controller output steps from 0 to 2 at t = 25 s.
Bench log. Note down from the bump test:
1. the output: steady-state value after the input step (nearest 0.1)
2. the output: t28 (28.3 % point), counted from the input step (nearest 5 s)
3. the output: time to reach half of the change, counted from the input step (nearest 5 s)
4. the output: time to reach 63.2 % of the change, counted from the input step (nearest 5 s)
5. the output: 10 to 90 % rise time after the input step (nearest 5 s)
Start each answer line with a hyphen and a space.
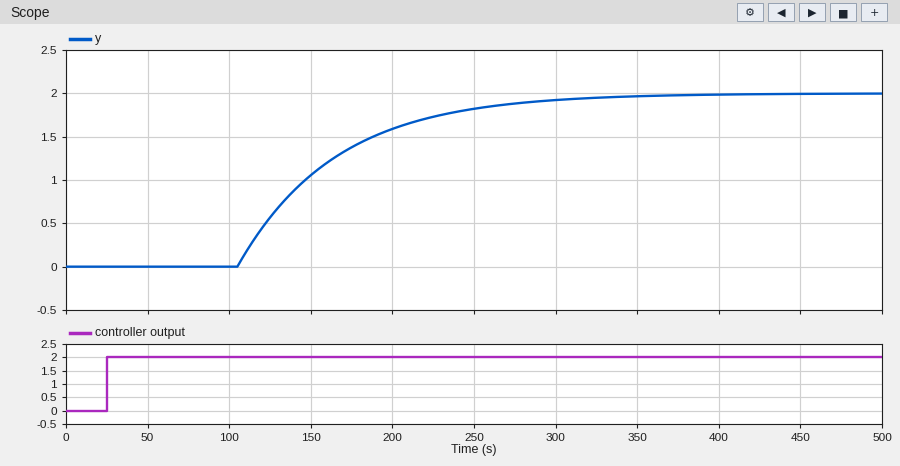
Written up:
- 2.0
- 100 s
- 120 s
- 140 s
- 130 s
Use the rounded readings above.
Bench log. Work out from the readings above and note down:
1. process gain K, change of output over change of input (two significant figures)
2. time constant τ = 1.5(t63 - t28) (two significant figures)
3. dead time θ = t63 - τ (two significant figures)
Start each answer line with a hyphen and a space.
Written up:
- 1.0
- 60 s
- 80 s
